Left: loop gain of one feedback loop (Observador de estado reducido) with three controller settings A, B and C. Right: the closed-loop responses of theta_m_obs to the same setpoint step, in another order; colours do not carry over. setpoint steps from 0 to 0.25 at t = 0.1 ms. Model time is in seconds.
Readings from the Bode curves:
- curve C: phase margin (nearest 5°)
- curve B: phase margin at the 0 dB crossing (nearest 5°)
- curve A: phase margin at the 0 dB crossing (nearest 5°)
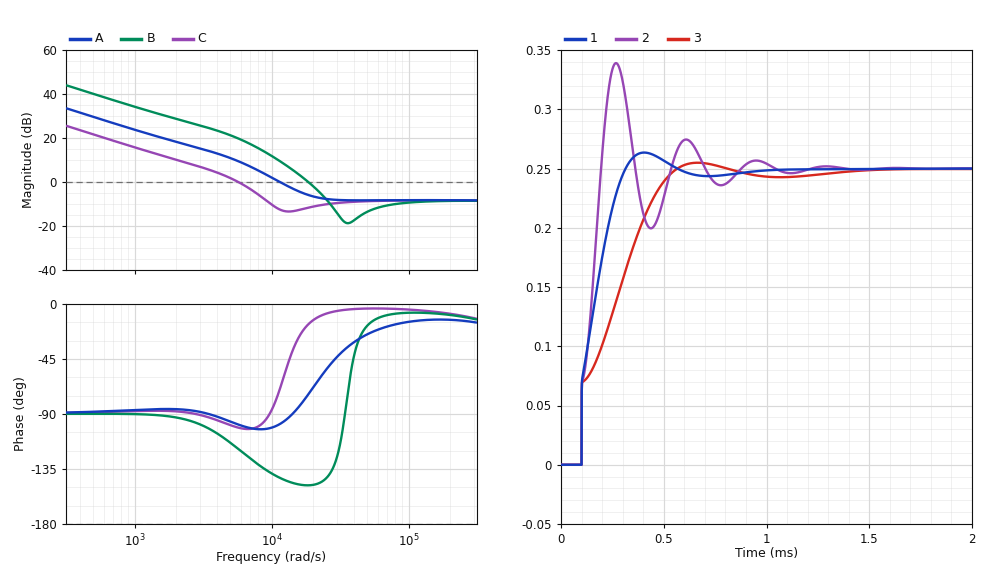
80°
30°
80°
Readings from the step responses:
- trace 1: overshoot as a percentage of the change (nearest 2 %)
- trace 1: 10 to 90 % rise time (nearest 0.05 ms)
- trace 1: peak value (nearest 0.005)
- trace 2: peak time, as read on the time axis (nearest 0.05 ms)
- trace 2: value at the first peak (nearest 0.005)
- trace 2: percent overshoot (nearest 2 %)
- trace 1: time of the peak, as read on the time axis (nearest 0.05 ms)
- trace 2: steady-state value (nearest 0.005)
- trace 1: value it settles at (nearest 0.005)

6 %
0.15 ms
0.265
0.25 ms
0.340
36 %
0.40 ms
0.250
0.250
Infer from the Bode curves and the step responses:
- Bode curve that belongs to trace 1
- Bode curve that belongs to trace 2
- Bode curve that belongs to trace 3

A
B
C
